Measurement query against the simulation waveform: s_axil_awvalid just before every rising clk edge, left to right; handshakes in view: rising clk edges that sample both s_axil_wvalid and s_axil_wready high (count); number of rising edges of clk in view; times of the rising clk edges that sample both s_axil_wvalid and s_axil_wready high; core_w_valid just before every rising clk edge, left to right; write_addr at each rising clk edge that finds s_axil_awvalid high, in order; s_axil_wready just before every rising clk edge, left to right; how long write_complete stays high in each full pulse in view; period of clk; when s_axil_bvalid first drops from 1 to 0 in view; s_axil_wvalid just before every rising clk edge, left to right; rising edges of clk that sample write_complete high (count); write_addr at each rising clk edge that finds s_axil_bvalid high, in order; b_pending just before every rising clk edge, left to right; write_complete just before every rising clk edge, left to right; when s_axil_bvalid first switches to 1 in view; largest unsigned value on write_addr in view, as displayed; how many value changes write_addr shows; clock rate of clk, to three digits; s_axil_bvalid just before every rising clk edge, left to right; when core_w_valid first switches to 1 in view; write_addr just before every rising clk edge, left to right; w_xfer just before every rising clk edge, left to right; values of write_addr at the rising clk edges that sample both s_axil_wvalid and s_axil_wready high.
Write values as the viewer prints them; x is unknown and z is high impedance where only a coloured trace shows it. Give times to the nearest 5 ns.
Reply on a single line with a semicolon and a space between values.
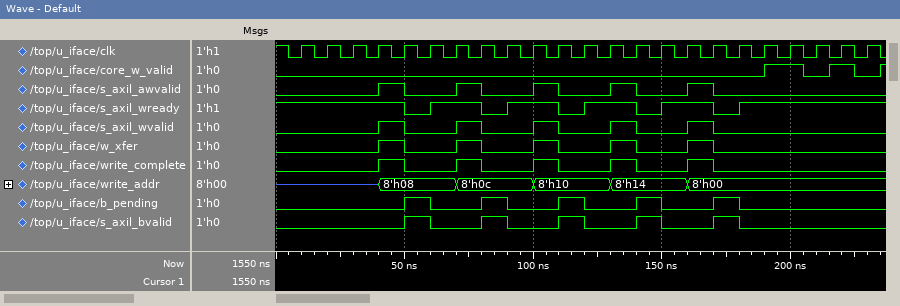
0 0 0 0 1 0 0 1 0 0 1 0 0 1 0 0 1 0 0 0 0 0 0; 5; 23; 50 ns, 80 ns, 110 ns, 140 ns, 170 ns; 0 0 0 0 0 0 0 0 0 0 0 0 0 0 0 0 0 0 0 1 0 1 0; 8'h08, 8'h0c, 8'h10, 8'h14, 8'h00; 1 1 1 1 1 0 1 1 0 1 1 0 1 1 0 1 1 0 1 1 1 1 1; 10 ns, 10 ns, 10 ns, 10 ns, 10 ns; 10 ns; 60 ns; 0 0 0 0 1 0 0 1 0 0 1 0 0 1 0 0 1 0 0 0 0 0 0; 5; 8'h08, 8'h0c, 8'h10, 8'h14, 8'h00; 0 0 0 0 0 1 0 0 1 0 0 1 0 0 1 0 0 1 0 0 0 0 0; 0 0 0 0 1 0 0 1 0 0 1 0 0 1 0 0 1 0 0 0 0 0 0; 50 ns; 8'h14; 5; 100 MHz; 0 0 0 0 0 1 0 0 1 0 0 1 0 0 1 0 0 1 0 0 0 0 0; 190 ns; z, z, z, z, 8'h08, 8'h08, 8'h08, 8'h0c, 8'h0c, 8'h0c, 8'h10, 8'h10, 8'h10, 8'h14, 8'h14, 8'h14, 8'h00, 8'h00, 8'h00, 8'h00, 8'h00, 8'h00, 8'h00; 0 0 0 0 1 0 0 1 0 0 1 0 0 1 0 0 1 0 0 0 0 0 0; 8'h08, 8'h0c, 8'h10, 8'h14, 8'h00
